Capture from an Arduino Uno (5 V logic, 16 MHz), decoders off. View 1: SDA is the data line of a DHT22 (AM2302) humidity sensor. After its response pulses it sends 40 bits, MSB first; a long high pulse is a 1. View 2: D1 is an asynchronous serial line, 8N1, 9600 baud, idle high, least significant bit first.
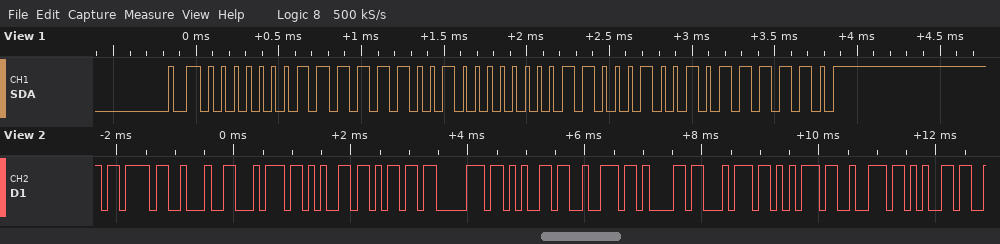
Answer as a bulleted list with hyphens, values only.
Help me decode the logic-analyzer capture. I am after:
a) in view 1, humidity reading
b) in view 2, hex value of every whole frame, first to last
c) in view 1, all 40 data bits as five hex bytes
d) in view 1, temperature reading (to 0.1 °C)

- 50.5 %
- 7B 22 74 65 6D 70 65 72 61 74 75 72 65
- 01 F9 00 C4 BE
- 19.6 °C
